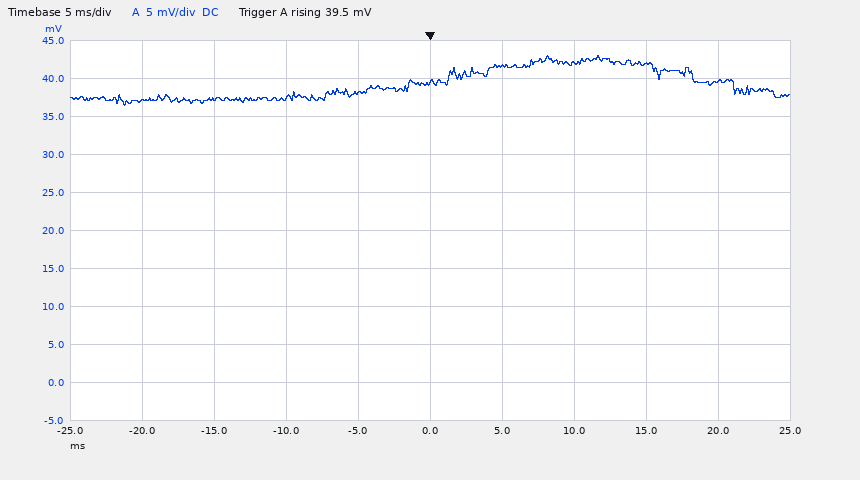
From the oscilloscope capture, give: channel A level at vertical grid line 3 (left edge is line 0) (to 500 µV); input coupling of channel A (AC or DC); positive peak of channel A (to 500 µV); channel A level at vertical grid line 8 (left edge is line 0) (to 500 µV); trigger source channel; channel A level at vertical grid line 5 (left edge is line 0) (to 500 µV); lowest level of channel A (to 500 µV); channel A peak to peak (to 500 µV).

37.5 mV
DC
43.0 mV
42.0 mV
channel A
39.5 mV
36.5 mV
6.5 mV
